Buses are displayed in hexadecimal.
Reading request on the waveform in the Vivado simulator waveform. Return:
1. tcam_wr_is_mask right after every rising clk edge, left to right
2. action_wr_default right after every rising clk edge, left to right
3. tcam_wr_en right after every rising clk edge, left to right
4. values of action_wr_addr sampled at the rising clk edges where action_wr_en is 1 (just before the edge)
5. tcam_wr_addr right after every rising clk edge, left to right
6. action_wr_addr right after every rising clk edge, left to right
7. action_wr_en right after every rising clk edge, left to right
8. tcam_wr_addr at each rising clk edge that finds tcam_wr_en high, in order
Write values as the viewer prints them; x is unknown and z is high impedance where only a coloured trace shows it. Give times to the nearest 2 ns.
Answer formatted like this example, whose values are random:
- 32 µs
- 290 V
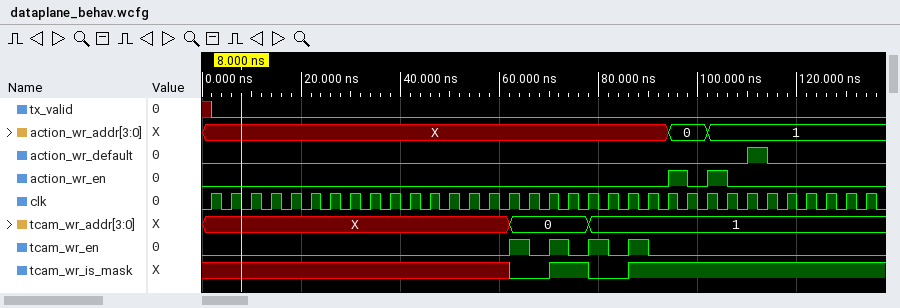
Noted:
- x x x x x x x x x x x x x x x 0 0 1 1 0 0 1 1 1 1 1 1 1 1 1 1 1 1 1
- 0 0 0 0 0 0 0 0 0 0 0 0 0 0 0 0 0 0 0 0 0 0 0 0 0 0 0 1 0 0 0 0 0 0
- 0 0 0 0 0 0 0 0 0 0 0 0 0 0 0 1 0 1 0 1 0 1 0 0 0 0 0 0 0 0 0 0 0 0
- 0, 1
- X, X, X, X, X, X, X, X, X, X, X, X, X, X, X, 0, 0, 0, 0, 1, 1, 1, 1, 1, 1, 1, 1, 1, 1, 1, 1, 1, 1, 1
- X, X, X, X, X, X, X, X, X, X, X, X, X, X, X, X, X, X, X, X, X, X, X, 0, 0, 1, 1, 1, 1, 1, 1, 1, 1, 1
- 0 0 0 0 0 0 0 0 0 0 0 0 0 0 0 0 0 0 0 0 0 0 0 1 0 1 0 0 0 0 0 0 0 0
- 0, 0, 1, 1
